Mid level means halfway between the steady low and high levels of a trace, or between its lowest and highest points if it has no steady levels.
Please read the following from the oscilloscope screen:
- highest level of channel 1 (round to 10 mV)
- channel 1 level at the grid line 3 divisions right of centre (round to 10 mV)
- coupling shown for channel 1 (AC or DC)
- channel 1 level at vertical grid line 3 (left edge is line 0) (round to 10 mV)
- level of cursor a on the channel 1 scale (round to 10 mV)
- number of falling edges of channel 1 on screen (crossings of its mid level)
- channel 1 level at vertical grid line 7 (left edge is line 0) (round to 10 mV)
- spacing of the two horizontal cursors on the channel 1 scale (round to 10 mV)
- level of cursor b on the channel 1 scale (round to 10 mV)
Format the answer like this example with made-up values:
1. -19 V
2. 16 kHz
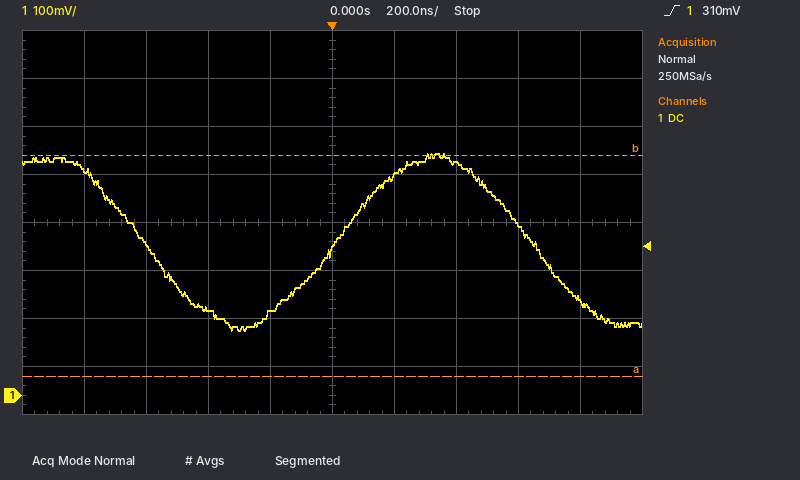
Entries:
1. 500 mV
2. 360 mV
3. DC
4. 180 mV
5. 40 mV
6. 2
7. 480 mV
8. 460 mV
9. 500 mV
